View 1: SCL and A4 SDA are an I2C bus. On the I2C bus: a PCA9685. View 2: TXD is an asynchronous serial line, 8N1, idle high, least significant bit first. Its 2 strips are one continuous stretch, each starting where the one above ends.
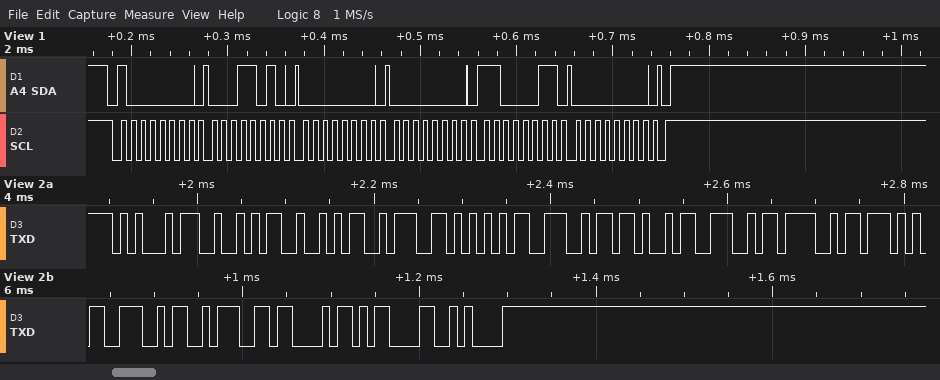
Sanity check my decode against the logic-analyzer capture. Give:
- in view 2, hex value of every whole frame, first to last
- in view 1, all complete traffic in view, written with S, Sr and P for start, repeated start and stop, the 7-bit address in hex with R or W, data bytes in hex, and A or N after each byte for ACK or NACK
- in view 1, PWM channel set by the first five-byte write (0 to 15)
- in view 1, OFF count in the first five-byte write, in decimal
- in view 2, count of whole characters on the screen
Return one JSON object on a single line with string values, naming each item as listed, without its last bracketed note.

{"in view 2, hex value of every whole frame, first to last": "45 52 52 3A 55 4E 4B 4E 4F 57 4E 3A 43 0D 0A", "in view 1, all complete traffic in view, written with S, Sr and P for start, repeated start and stop, the 7-bit address in hex with R or W, data bytes in hex, and A or N after each byte for ACK or NACK": "S 40W A 1A A 00 A 00 A C3 A 00 A P", "in view 1, PWM channel set by the first five-byte write": "5", "in view 1, OFF count in the first five-byte write, in decimal": "195", "in view 2, count of whole characters on the screen": "15"}
